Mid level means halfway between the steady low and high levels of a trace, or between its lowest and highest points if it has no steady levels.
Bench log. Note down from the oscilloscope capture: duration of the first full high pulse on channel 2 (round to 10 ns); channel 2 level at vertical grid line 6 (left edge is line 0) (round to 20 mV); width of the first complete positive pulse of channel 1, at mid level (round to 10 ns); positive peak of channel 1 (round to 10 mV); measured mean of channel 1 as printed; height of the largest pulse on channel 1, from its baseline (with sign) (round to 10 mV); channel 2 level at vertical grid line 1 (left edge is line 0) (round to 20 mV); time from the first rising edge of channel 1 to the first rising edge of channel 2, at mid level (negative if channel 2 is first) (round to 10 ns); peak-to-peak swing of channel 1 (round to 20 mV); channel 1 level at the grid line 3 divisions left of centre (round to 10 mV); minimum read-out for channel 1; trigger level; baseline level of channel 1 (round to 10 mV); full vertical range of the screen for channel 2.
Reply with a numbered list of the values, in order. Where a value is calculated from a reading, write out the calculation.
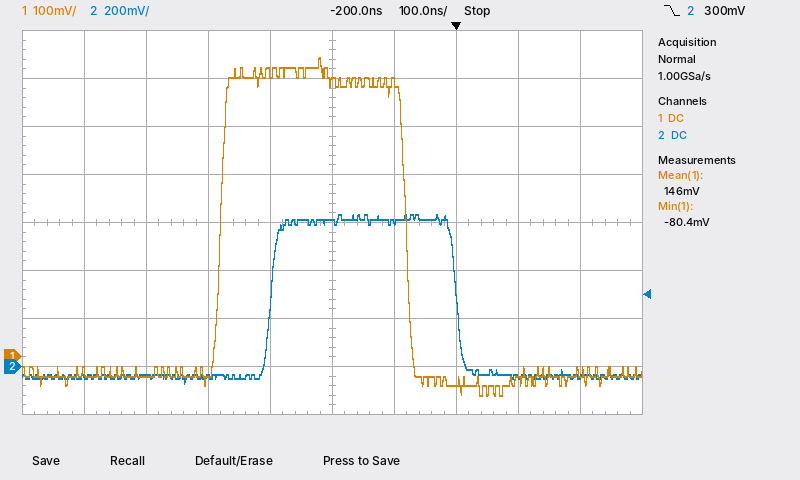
1. 300 ns
2. 600 mV
3. 300 ns
4. 620 mV
5. 146 mV
6. 620 mV − (-40 mV) = +660 mV
7. -40 mV
8. +80 ns
9. 700 mV
10. -40 mV
11. -80.4 mV
12. 300 mV
13. -40 mV
14. 1.6 V
